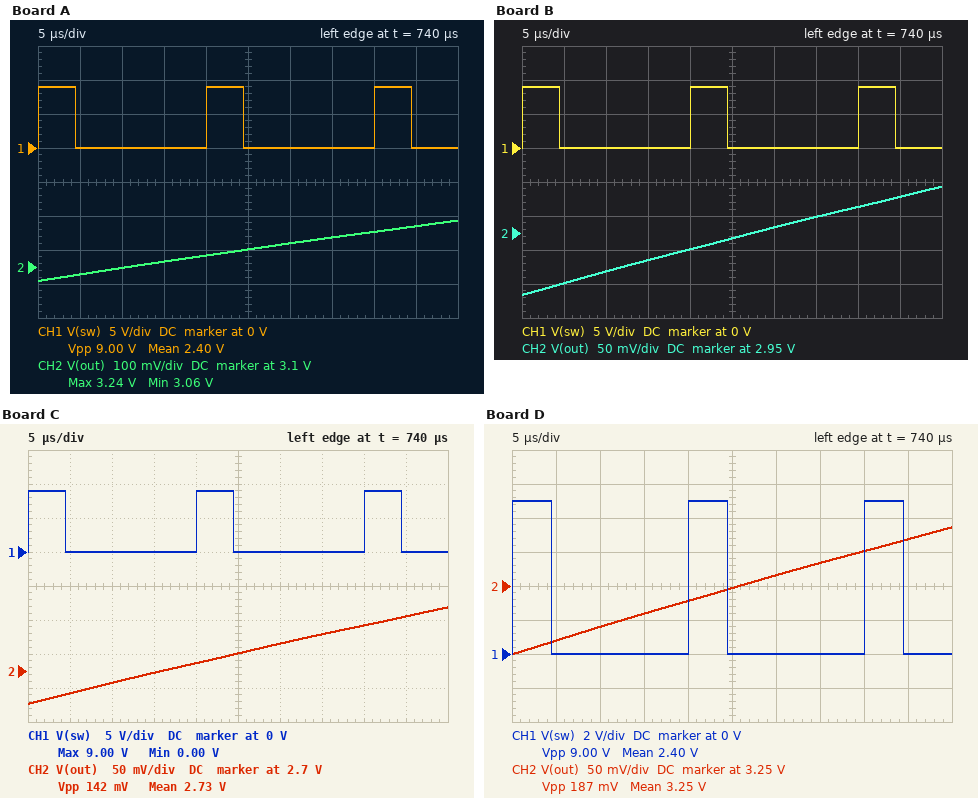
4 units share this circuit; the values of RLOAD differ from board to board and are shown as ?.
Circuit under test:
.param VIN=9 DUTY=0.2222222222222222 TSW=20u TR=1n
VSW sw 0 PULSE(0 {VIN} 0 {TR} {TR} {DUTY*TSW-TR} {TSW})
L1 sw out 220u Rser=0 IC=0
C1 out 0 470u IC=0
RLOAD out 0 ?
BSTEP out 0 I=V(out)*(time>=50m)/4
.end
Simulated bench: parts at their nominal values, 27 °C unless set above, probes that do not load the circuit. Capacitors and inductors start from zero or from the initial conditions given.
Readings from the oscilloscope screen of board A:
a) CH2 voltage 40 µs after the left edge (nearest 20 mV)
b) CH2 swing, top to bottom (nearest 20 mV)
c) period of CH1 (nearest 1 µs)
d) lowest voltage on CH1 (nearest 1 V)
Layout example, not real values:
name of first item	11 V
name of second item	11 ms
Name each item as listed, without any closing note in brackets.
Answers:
CH2 voltage 40 µs after the left edge	3.20 V
CH2 swing, top to bottom	180 mV
period of CH1	20 µs
lowest voltage on CH1	0 V
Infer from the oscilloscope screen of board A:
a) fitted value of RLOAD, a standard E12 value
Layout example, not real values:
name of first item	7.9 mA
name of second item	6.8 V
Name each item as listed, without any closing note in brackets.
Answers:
fitted value of RLOAD, a standard E12 value	4.7 Ω
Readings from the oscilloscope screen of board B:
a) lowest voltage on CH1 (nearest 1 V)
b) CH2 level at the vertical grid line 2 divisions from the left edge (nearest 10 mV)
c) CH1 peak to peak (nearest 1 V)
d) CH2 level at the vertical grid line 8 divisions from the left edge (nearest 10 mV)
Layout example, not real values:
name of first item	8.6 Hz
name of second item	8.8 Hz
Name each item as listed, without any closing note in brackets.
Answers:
lowest voltage on CH1	0 V
CH2 level at the vertical grid line 2 divisions from the left edge	2.89 V
CH1 peak to peak	9 V
CH2 level at the vertical grid line 8 divisions from the left edge	2.99 V
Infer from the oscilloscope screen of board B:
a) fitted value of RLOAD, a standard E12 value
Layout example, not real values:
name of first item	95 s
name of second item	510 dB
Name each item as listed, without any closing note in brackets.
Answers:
fitted value of RLOAD, a standard E12 value	2.7 Ω
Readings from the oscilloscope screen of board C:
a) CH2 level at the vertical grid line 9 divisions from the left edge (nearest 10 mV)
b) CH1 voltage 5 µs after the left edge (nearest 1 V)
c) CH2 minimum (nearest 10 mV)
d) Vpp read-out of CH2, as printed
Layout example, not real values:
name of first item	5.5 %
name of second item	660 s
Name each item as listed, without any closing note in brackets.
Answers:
CH2 level at the vertical grid line 9 divisions from the left edge	2.78 V
CH1 voltage 5 µs after the left edge	0 V
CH2 minimum	2.65 V
Vpp read-out of CH2, as printed	142 mV
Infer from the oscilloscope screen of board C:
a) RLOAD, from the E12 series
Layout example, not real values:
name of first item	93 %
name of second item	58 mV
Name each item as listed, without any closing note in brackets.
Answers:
RLOAD, from the E12 series	1.8 Ω
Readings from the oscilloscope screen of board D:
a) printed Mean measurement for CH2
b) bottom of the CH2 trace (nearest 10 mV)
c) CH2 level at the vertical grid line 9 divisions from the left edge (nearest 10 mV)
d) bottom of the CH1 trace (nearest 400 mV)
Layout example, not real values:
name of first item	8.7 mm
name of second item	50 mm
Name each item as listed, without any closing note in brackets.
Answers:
printed Mean measurement for CH2	3.25 V
bottom of the CH2 trace	3.15 V
CH2 level at the vertical grid line 9 divisions from the left edge	3.32 V
bottom of the CH1 trace	0 V
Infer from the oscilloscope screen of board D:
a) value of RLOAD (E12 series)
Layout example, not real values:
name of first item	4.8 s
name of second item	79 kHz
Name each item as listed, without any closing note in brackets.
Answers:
value of RLOAD	6.8 Ω
